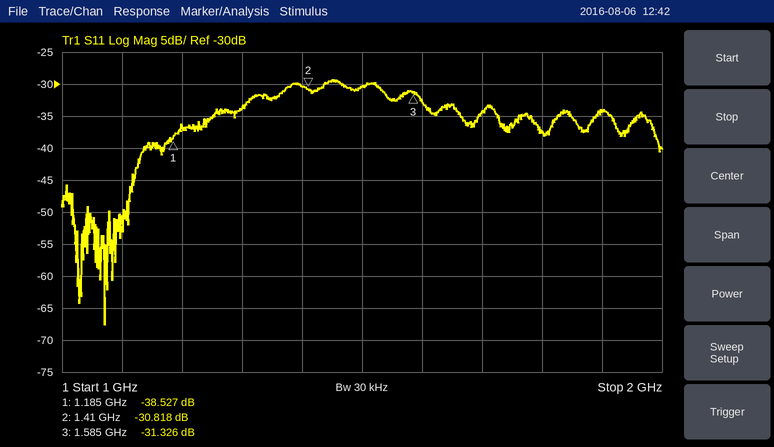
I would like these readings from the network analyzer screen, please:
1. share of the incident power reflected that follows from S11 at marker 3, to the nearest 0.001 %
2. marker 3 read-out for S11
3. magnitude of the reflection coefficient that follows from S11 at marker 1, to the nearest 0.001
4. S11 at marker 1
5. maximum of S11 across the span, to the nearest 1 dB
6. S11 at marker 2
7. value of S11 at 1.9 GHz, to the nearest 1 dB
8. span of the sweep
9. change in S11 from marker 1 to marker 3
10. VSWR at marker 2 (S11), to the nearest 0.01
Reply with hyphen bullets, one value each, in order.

- 0.074 %
- -31.326 dB
- 0.012
- -38.527 dB
- -29 dB
- -30.818 dB
- -34 dB
- 1 GHz
- 7.201 dB
- 1.06
